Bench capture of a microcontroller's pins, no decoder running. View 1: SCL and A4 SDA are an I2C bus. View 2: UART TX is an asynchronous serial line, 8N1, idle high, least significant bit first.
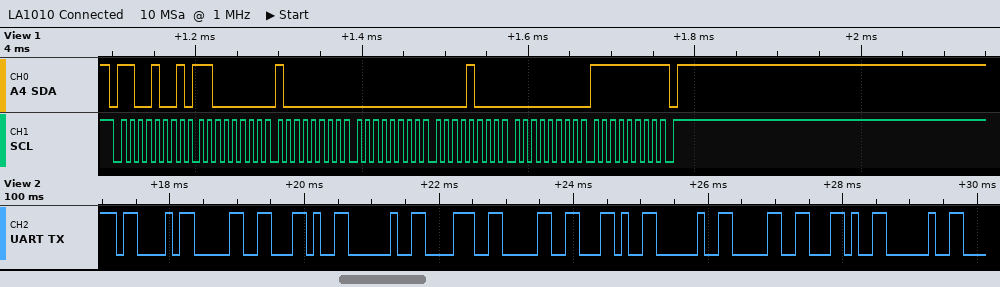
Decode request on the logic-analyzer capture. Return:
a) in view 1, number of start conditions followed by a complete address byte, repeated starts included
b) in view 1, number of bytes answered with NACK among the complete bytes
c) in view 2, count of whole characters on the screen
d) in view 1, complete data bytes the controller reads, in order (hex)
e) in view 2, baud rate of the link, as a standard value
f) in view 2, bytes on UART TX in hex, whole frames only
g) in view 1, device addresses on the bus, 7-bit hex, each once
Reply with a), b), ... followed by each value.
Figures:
a) 1
b) 1
c) 11
d) C0 80 00 08 00 FF
e) 9600 baud
f) 43 30 2C 20 38 30 2C 20 30 2C 20
g) 0x64
